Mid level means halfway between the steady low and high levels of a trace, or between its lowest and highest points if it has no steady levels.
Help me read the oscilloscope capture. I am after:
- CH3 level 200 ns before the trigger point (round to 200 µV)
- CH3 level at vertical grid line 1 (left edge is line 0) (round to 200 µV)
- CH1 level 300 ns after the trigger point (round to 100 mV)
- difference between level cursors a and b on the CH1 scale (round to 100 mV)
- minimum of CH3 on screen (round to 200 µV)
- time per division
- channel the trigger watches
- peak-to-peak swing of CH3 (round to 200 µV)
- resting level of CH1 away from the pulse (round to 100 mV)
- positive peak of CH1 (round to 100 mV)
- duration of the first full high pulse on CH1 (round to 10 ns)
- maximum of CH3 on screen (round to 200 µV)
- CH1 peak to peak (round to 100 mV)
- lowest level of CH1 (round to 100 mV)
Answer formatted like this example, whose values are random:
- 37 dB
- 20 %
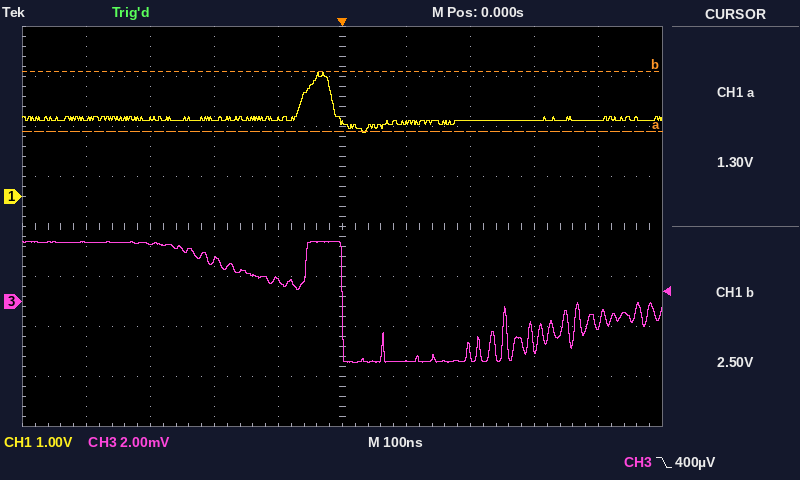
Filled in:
- 1.6 mV
- 2.4 mV
- 1.5 V
- 1.2 V
- -2.4 mV
- 100 ns
- CH3
- 4.8 mV
- 1.5 V
- 2.5 V
- 50 ns
- 2.4 mV
- 1.2 V
- 1.3 V
